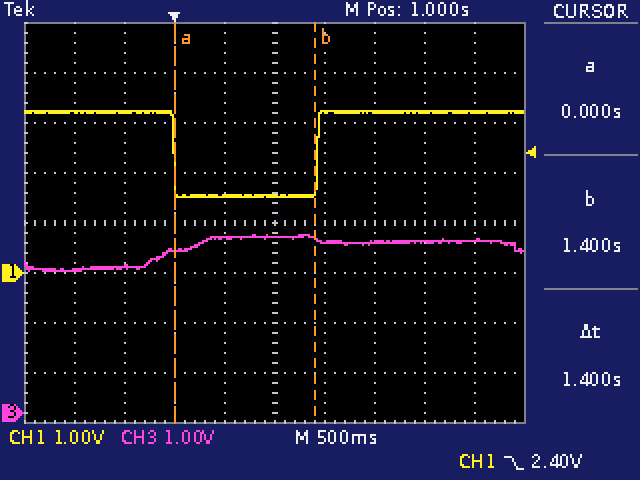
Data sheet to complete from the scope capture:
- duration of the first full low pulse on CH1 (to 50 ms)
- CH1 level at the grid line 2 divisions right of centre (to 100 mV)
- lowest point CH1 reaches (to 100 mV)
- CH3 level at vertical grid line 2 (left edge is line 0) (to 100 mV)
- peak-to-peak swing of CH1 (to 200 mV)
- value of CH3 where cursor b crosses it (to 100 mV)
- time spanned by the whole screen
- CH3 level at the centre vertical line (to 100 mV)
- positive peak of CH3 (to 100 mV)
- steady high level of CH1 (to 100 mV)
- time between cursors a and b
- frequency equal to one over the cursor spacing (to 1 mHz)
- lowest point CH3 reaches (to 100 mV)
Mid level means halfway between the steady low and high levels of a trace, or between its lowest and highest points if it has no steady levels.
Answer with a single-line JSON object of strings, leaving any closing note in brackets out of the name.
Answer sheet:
{"duration of the first full low pulse on CH1": "1.45 s", "CH1 level at the grid line 2 divisions right of centre": "3.2 V", "lowest point CH1 reaches": "1.5 V", "CH3 level at vertical grid line 2 (left edge is line 0)": "2.9 V", "peak-to-peak swing of CH1": "1.8 V", "value of CH3 where cursor b crosses it": "3.5 V", "time spanned by the whole screen": "5 s", "CH3 level at the centre vertical line": "3.5 V", "positive peak of CH3": "3.6 V", "steady high level of CH1": "3.2 V", "time between cursors a and b": "1.4 s", "frequency equal to one over the cursor spacing": "714 mHz", "lowest point CH3 reaches": "2.8 V"}
